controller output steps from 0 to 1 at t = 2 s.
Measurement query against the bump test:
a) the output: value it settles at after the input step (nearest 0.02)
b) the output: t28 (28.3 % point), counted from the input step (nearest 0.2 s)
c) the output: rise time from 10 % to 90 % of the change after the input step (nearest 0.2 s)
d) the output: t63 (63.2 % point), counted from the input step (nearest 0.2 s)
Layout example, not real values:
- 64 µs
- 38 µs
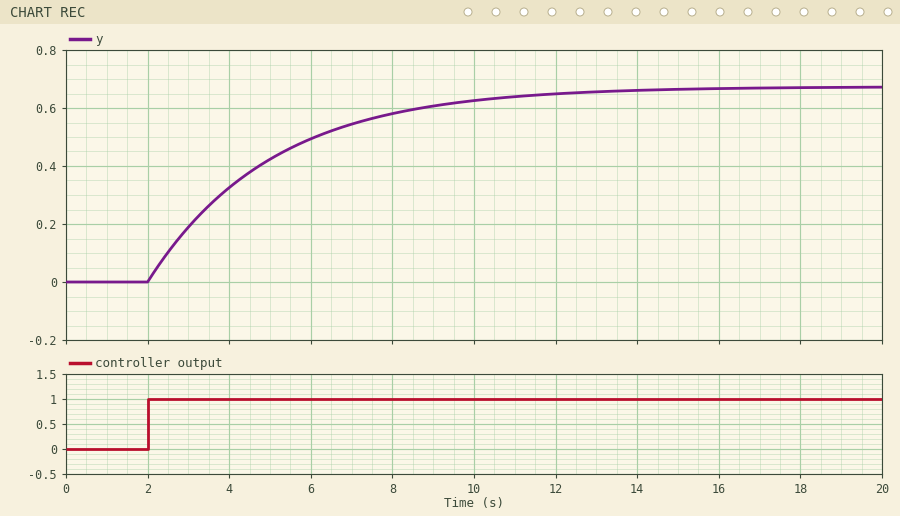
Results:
- 0.68
- 1.0 s
- 6.6 s
- 3.0 s
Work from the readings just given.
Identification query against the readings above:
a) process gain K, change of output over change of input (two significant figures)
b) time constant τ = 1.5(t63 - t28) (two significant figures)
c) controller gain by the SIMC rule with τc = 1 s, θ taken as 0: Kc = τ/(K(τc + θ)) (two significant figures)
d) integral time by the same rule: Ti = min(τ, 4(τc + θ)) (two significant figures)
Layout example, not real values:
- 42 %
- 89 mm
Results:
- 0.68
- 3.0 s
- 4.4
- 3.0 s
